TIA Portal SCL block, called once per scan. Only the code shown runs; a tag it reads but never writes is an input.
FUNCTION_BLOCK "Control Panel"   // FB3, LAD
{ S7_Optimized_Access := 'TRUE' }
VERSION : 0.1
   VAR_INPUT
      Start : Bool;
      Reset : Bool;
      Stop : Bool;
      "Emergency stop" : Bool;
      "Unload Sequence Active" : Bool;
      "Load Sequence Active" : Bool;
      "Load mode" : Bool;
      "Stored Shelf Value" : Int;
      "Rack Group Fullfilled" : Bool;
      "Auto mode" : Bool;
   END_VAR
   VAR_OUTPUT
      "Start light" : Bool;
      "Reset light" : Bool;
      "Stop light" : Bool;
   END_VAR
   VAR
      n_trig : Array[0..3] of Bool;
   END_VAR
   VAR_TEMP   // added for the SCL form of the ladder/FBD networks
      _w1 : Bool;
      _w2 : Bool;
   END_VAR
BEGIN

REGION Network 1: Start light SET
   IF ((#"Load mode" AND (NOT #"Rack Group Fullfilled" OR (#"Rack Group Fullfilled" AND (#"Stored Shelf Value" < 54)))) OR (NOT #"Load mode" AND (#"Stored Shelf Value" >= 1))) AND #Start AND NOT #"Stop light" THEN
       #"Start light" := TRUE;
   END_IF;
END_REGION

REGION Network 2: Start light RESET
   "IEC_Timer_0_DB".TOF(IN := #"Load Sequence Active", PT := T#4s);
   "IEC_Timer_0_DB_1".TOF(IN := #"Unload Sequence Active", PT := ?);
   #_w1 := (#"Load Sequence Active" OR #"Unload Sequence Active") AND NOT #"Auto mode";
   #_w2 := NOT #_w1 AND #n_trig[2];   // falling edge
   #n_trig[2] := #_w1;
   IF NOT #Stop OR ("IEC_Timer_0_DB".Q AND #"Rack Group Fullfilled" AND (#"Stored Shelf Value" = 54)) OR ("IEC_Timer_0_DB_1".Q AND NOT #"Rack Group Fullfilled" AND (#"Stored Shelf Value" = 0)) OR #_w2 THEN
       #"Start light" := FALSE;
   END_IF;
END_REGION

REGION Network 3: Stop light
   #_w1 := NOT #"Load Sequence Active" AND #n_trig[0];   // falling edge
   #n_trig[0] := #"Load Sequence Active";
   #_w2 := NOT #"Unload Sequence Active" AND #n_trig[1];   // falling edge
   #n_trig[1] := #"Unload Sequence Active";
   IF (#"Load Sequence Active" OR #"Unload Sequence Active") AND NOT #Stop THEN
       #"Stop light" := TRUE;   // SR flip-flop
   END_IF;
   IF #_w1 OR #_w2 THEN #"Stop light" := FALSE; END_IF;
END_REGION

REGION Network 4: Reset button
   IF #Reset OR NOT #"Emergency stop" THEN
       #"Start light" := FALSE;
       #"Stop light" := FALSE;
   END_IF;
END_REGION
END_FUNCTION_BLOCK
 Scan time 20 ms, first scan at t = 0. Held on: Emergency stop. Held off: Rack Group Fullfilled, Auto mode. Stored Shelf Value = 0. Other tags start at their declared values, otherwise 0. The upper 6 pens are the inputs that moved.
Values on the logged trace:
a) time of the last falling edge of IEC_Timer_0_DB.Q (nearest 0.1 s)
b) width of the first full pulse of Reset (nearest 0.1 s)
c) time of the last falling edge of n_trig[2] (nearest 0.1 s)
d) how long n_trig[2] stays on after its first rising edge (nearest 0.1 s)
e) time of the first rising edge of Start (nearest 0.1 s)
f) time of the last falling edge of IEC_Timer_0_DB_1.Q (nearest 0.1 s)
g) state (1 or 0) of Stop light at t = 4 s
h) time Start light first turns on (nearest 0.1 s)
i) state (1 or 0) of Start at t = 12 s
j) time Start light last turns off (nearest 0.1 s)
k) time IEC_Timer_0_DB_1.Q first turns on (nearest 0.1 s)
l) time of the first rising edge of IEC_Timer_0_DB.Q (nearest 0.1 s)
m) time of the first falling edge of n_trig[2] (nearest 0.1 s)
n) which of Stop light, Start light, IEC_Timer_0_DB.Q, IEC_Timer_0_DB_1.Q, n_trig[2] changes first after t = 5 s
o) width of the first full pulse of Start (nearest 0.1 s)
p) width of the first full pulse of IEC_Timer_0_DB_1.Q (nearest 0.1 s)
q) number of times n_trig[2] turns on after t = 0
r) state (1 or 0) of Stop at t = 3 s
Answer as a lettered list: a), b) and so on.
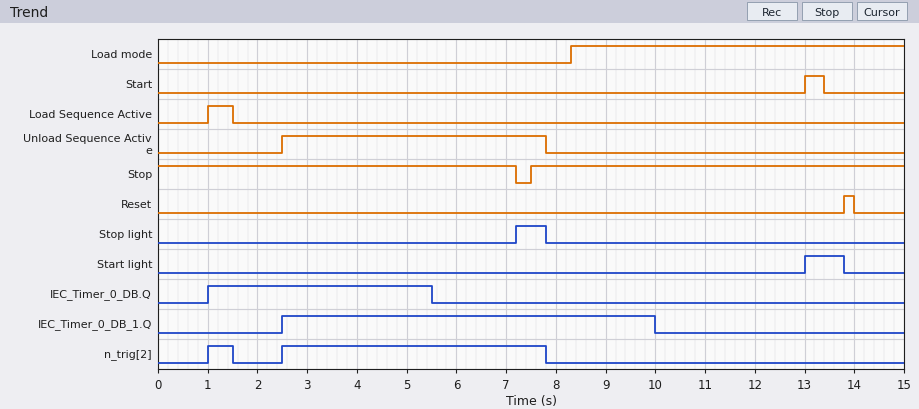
a) 5.5 s
b) 0.2 s
c) 7.8 s
d) 0.5 s
e) 13.0 s
f) 10.0 s
g) 0
h) 13.0 s
i) 0
j) 13.8 s
k) 2.5 s
l) 1.0 s
m) 1.5 s
n) IEC_Timer_0_DB.Q
o) 0.4 s
p) 7.5 s
q) 2
r) 1
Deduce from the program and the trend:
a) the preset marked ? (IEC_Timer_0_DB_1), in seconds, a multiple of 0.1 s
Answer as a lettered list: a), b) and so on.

a) 2.2 s
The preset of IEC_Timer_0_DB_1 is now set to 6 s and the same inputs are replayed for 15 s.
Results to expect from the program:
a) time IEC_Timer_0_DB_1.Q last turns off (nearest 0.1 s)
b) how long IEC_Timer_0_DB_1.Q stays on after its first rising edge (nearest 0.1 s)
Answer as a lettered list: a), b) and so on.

a) 13.8 s
b) 11.3 s
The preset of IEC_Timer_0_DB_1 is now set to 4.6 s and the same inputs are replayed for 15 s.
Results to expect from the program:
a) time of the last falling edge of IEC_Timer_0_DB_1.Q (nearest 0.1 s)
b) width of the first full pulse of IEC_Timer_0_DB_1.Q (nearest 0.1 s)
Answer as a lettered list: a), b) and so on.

a) 12.4 s
b) 9.9 s
